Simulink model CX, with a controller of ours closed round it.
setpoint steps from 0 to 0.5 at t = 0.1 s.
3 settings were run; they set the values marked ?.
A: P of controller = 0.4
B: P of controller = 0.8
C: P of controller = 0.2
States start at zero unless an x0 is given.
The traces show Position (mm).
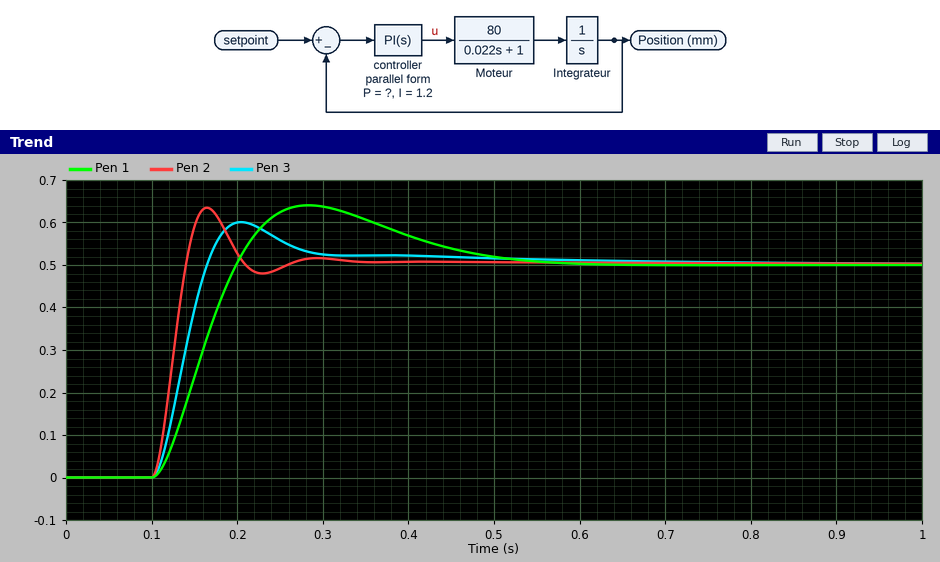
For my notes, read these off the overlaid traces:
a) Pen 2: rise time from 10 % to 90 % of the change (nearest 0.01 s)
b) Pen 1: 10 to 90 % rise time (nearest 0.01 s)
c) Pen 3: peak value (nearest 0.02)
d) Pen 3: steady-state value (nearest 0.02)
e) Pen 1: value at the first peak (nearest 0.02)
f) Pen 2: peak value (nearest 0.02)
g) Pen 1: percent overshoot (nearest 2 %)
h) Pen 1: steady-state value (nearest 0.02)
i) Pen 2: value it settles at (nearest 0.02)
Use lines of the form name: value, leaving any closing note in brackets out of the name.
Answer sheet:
Pen 2: rise time from 10 % to 90 % of the change: 0.03 s
Pen 1: 10 to 90 % rise time: 0.07 s
Pen 3: peak value: 0.60
Pen 3: steady-state value: 0.50
Pen 1: value at the first peak: 0.64
Pen 2: peak value: 0.64
Pen 1: percent overshoot: 28 %
Pen 1: steady-state value: 0.50
Pen 2: value it settles at: 0.50
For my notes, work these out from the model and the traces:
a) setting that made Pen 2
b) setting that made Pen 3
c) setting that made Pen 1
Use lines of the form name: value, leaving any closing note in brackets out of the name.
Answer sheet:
setting that made Pen 2: B
setting that made Pen 3: A
setting that made Pen 1: C
